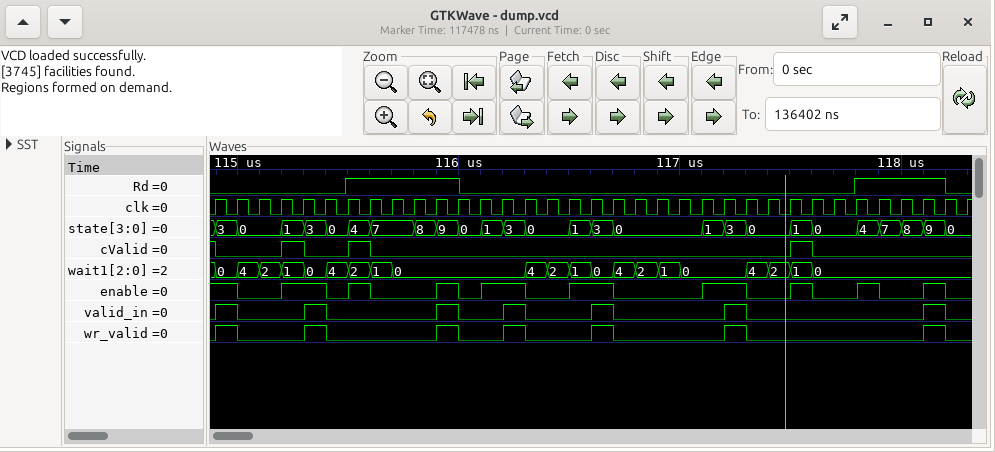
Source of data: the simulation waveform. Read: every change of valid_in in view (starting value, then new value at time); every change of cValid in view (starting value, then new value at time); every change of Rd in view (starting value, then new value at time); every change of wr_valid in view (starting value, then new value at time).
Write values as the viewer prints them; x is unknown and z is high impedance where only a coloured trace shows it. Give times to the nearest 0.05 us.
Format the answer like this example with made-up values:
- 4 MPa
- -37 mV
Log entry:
- 0, 1 at 114.9 us, 0 at 115 us, 1 at 115.3 us, 0 at 115.4 us, 1 at 115.9 us, 0 at 116 us, 1 at 116.2 us, 0 at 116.3 us, 1 at 116.6 us, 0 at 116.7 us, 1 at 117.2 us, 0 at 117.3 us, 1 at 118.1 us, 0 at 118.2 us
- 1, 0 at 114.9 us, 1 at 115.2 us, 0 at 115.3 us, 1 at 115.5 us, 0 at 115.6 us, 1 at 117.5 us, 0 at 117.6 us
- 0, 1 at 115.5 us, 0 at 116 us, 1 at 117.8 us, 0 at 118.2 us
- 0, 1 at 114.9 us, 0 at 115 us, 1 at 115.3 us, 0 at 115.4 us, 1 at 115.9 us, 0 at 116 us, 1 at 116.2 us, 0 at 116.3 us, 1 at 116.6 us, 0 at 116.7 us, 1 at 117.2 us, 0 at 117.3 us, 1 at 118.1 us, 0 at 118.2 us
